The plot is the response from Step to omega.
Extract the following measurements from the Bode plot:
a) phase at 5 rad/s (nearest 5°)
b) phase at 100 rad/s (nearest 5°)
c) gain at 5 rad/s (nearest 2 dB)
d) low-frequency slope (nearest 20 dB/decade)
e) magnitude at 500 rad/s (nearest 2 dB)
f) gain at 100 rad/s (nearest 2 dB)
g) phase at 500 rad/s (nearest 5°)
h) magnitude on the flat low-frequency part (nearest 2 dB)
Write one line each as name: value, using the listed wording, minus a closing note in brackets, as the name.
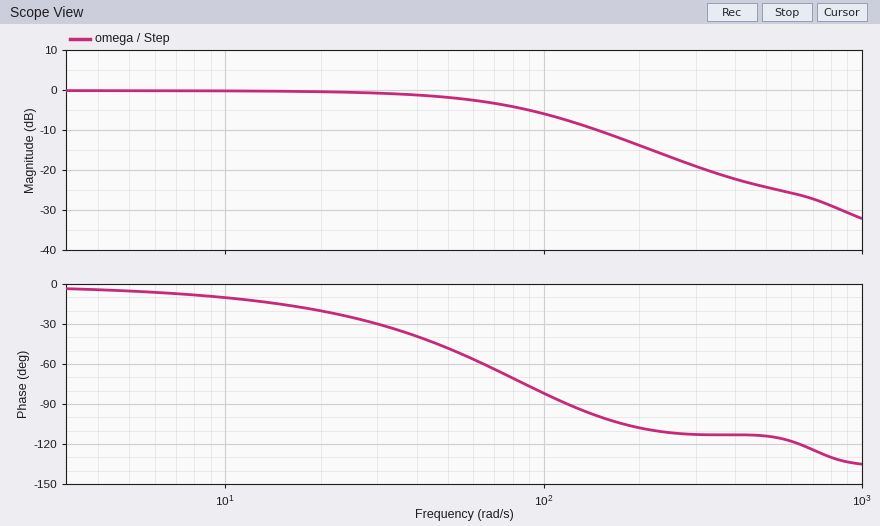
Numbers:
phase at 5 rad/s: -5°
phase at 100 rad/s: -80°
gain at 5 rad/s: 0 dB
low-frequency slope: 0 dB/decade
magnitude at 500 rad/s: -24 dB
gain at 100 rad/s: -6 dB
phase at 500 rad/s: -115°
magnitude on the flat low-frequency part: 0 dB
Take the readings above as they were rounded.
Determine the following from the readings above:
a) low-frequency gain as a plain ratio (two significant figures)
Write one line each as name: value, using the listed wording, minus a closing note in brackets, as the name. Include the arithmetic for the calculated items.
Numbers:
low-frequency gain as a plain ratio: 10^(0 / 20) = 1.0
